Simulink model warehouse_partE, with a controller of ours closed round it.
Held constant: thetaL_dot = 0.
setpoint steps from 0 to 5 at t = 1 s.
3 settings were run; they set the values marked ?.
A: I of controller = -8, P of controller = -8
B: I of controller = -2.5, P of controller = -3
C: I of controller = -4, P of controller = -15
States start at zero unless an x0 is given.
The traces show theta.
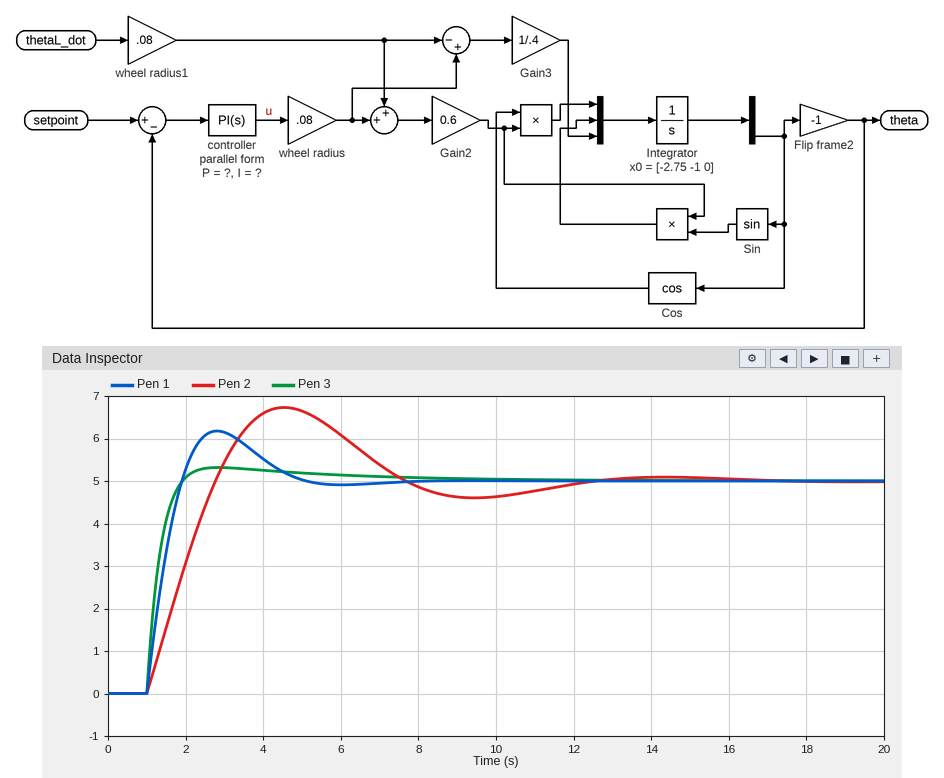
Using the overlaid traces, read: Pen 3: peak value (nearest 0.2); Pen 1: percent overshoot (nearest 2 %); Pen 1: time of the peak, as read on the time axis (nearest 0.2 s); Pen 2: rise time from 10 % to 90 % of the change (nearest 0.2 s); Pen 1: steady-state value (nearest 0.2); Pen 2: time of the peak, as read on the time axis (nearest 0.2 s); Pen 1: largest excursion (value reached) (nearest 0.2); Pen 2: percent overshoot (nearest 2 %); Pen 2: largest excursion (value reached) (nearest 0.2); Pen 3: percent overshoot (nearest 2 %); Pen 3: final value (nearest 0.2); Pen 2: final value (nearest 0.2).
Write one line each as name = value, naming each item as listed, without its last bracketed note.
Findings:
Pen 3: peak value = 5.4
Pen 1: percent overshoot = 24 %
Pen 1: time of the peak, as read on the time axis = 2.8 s
Pen 2: rise time from 10 % to 90 % of the change = 1.4 s
Pen 1: steady-state value = 5.0
Pen 2: time of the peak, as read on the time axis = 4.6 s
Pen 1: largest excursion (value reached) = 6.2
Pen 2: percent overshoot = 34 %
Pen 2: largest excursion (value reached) = 6.8
Pen 3: percent overshoot = 6 %
Pen 3: final value = 5.0
Pen 2: final value = 5.0
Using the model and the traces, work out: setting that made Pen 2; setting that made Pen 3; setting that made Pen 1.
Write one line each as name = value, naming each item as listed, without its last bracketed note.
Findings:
setting that made Pen 2 = B
setting that made Pen 3 = C
setting that made Pen 1 = A
